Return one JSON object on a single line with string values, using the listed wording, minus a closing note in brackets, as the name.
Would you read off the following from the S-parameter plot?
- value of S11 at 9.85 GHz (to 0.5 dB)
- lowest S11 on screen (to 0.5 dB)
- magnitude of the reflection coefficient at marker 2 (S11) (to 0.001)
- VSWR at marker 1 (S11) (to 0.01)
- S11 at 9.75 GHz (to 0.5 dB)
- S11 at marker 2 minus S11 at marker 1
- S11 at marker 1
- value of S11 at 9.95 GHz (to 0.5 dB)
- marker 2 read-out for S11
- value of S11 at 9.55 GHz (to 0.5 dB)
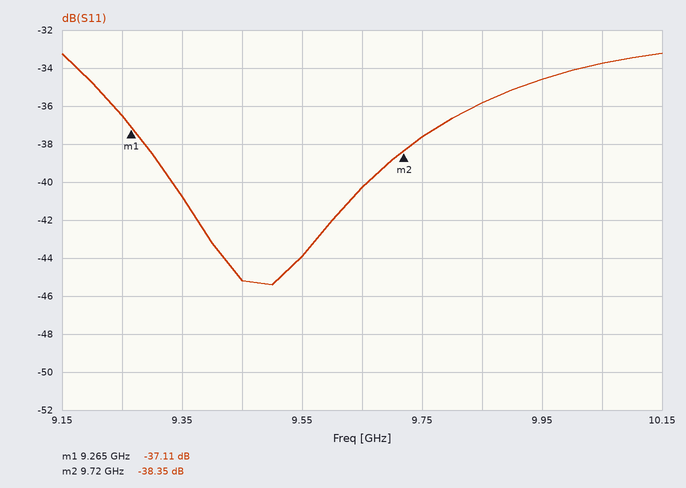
{"value of S11 at 9.85 GHz": "-36.0 dB", "lowest S11 on screen": "-45.5 dB", "magnitude of the reflection coefficient at marker 2 (S11)": "0.012", "VSWR at marker 1 (S11)": "1.03", "S11 at 9.75 GHz": "-37.5 dB", "S11 at marker 2 minus S11 at marker 1": "-1.24 dB", "S11 at marker 1": "-37.11 dB", "value of S11 at 9.95 GHz": "-34.5 dB", "marker 2 read-out for S11": "-38.35 dB", "value of S11 at 9.55 GHz": "-44.0 dB"}
